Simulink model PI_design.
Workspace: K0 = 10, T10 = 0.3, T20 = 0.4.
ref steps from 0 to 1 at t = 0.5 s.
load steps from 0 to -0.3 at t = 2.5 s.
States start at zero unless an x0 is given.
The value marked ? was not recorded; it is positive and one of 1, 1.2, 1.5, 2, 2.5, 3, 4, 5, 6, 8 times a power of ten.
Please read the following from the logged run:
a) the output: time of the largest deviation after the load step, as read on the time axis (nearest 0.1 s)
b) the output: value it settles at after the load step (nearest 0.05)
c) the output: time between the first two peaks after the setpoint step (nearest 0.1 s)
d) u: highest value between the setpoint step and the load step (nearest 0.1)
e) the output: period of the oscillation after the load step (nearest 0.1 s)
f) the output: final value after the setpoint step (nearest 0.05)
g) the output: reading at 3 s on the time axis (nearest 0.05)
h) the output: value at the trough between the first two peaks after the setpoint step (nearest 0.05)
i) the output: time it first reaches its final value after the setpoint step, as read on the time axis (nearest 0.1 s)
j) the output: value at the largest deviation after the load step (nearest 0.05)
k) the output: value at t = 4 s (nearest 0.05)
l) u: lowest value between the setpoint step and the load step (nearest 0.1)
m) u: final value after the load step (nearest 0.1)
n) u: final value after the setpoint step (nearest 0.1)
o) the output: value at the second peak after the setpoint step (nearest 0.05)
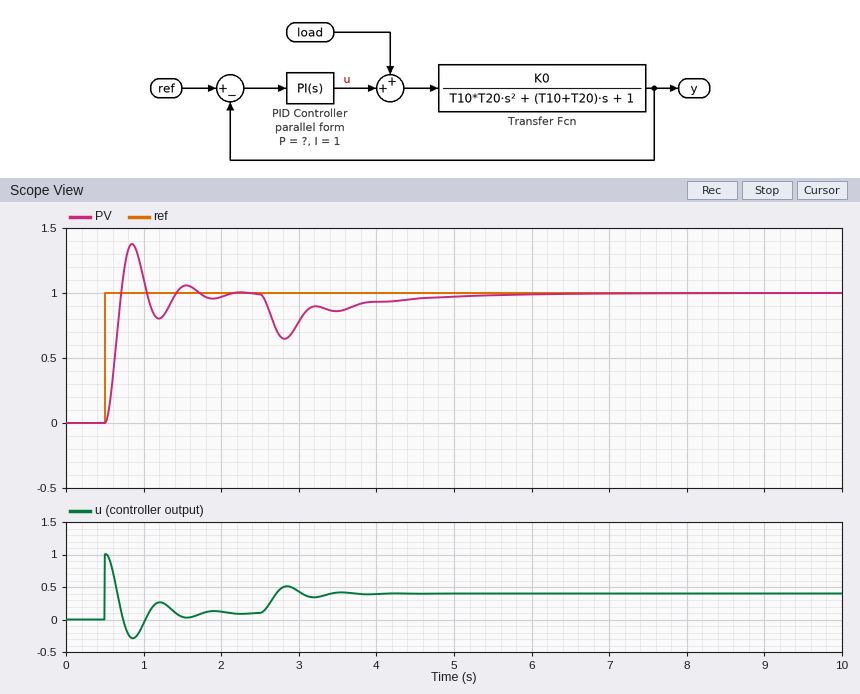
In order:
2.8 s
1.00
0.7 s
1.0
0.7 s
1.00
0.80
0.80
0.7 s
0.65
0.95
-0.3
0.4
0.1
1.05
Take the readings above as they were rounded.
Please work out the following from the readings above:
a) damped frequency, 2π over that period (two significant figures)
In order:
9.0 rad/s
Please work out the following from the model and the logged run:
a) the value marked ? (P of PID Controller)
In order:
1
